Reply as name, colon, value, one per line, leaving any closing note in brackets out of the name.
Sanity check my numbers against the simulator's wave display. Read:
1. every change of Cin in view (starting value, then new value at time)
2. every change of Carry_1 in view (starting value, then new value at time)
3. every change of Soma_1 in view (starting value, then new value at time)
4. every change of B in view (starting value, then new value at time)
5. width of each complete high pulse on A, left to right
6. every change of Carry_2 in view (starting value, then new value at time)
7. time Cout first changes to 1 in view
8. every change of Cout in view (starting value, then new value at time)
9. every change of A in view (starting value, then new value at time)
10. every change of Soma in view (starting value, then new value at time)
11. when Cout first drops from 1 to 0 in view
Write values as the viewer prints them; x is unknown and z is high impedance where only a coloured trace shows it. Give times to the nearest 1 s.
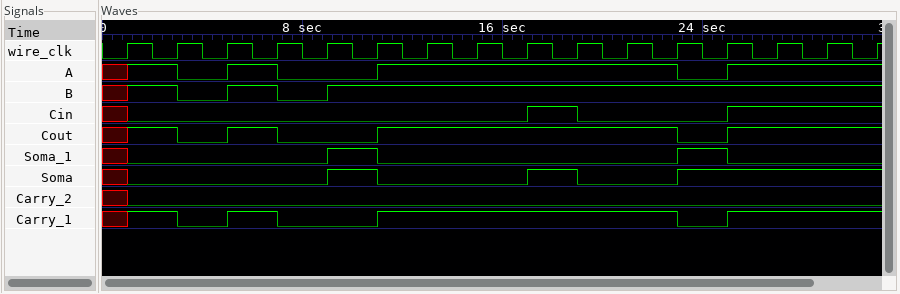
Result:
every change of Cin in view: x, 0 at 1 s, 1 at 17 s, 0 at 19 s, 1 at 25 s
every change of Carry_1 in view: x, 1 at 1 s, 0 at 3 s, 1 at 5 s, 0 at 7 s, 1 at 11 s, 0 at 23 s, 1 at 25 s
every change of Soma_1 in view: x, 0 at 1 s, 1 at 9 s, 0 at 11 s, 1 at 23 s, 0 at 25 s
every change of B in view: x, 1 at 1 s, 0 at 3 s, 1 at 5 s, 0 at 7 s, 1 at 9 s
width of each complete high pulse on A, left to right: 2 s, 12 s
every change of Carry_2 in view: x, 0 at 1 s
time Cout first changes to 1 in view: 1 s
every change of Cout in view: x, 1 at 1 s, 0 at 3 s, 1 at 5 s, 0 at 7 s, 1 at 11 s, 0 at 23 s, 1 at 25 s
every change of A in view: x, 1 at 1 s, 0 at 3 s, 1 at 5 s, 0 at 7 s, 1 at 11 s, 0 at 23 s, 1 at 25 s
every change of Soma in view: x, 0 at 1 s, 1 at 9 s, 0 at 11 s, 1 at 17 s, 0 at 19 s, 1 at 23 s
when Cout first drops from 1 to 0 in view: 3 s
